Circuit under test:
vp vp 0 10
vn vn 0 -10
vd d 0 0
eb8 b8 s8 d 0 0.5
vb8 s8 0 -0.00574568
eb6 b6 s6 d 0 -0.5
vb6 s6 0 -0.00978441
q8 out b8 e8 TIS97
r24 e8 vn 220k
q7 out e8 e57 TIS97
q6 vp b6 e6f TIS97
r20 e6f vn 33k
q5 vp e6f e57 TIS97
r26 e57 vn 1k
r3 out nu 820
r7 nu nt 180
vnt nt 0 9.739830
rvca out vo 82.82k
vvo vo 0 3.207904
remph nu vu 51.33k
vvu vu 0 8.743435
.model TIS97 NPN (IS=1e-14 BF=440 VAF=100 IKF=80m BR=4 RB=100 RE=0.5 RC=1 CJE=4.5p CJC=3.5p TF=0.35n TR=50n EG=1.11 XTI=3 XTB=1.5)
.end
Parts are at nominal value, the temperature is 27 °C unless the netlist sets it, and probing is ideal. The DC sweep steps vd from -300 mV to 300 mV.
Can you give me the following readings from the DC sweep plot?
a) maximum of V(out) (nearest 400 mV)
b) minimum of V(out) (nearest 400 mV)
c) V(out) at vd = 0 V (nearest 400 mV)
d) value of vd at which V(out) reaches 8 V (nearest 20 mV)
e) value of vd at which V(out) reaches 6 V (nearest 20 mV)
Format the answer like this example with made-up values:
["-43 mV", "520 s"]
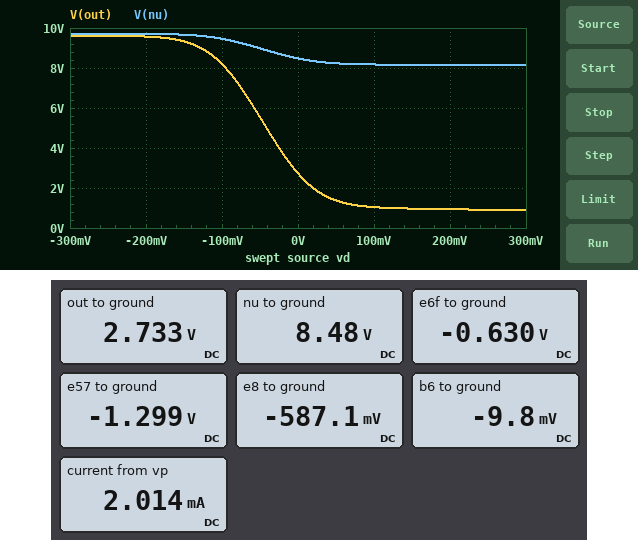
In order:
["9.6 V", "800 mV", "2.8 V", "-100 mV", "-60 mV"]
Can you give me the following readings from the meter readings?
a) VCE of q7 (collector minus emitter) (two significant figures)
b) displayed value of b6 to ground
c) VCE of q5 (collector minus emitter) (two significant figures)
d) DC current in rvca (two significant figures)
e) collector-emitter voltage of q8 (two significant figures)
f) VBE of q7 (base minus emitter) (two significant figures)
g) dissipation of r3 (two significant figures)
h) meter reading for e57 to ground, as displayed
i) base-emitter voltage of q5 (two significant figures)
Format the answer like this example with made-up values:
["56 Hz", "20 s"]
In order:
["4.0 V", "-9.8 mV", "11 V", "5.7 µA", "3.3 V", "710 mV", "40 mW", "-1.299 V", "670 mV"]
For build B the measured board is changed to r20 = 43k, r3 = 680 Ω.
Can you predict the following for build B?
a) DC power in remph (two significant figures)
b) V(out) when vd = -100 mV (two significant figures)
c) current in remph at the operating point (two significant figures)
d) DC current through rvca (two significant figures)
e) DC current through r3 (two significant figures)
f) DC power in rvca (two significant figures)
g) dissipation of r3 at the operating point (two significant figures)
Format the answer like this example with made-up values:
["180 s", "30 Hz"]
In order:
["900 nW", "8.6 V", "4.2 µA", "8.9 µA", "6.7 mA", "6.6 µW", "31 mW"]
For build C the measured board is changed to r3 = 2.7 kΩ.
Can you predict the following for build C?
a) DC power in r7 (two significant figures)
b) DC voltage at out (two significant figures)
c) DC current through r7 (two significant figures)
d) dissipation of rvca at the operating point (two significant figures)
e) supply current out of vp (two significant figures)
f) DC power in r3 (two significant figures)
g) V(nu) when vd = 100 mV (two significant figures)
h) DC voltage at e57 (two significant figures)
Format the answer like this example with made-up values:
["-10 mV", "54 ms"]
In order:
["2.3 mW", "-630 mV", "3.6 mA", "180 µW", "5.3 mA", "35 mW", "9.1 V", "-1.3 V"]
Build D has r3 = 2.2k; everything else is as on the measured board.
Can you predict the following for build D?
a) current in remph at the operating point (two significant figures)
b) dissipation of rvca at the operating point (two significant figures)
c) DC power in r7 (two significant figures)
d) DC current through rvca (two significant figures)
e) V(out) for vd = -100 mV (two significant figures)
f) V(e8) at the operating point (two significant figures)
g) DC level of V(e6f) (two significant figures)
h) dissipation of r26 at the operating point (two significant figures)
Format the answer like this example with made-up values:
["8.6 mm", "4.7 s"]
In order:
["4.1 µA", "180 µW", "3.4 mW", "46 µA", "6.2 V", "-630 mV", "-630 mV", "75 mW"]
